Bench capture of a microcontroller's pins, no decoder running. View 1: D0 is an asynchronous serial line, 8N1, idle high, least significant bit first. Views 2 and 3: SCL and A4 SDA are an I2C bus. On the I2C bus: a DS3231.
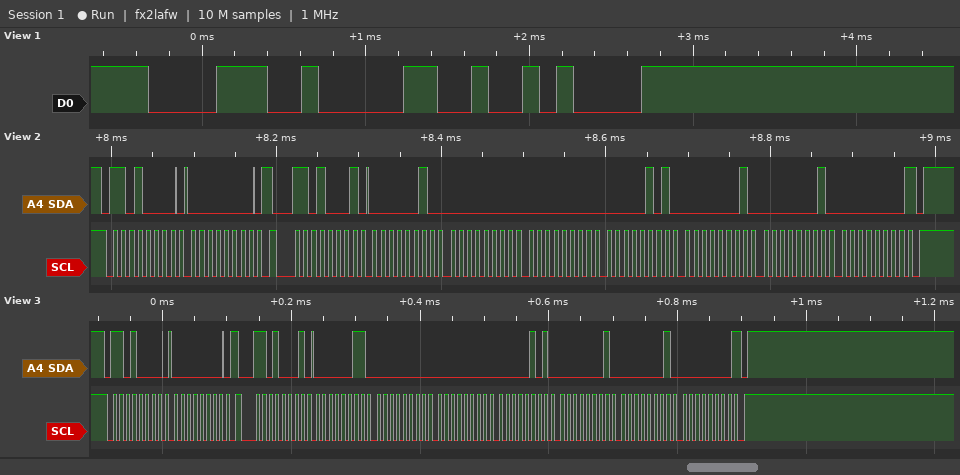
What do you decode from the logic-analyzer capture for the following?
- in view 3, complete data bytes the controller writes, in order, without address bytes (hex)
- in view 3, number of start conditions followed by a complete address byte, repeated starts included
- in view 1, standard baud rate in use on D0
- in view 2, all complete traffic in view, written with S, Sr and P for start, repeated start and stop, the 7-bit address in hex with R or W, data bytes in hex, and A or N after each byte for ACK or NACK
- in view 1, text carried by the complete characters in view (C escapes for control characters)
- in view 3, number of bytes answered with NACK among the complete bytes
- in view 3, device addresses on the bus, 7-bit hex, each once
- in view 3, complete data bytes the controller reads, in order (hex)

00
2
9600 baud
S 68W A 00 A Sr 68R A 02 A 00 A 00 A 05 A 01 A 01 A 00 N P
"80\n"
1
0x68
03 00 00 05 01 01 00
